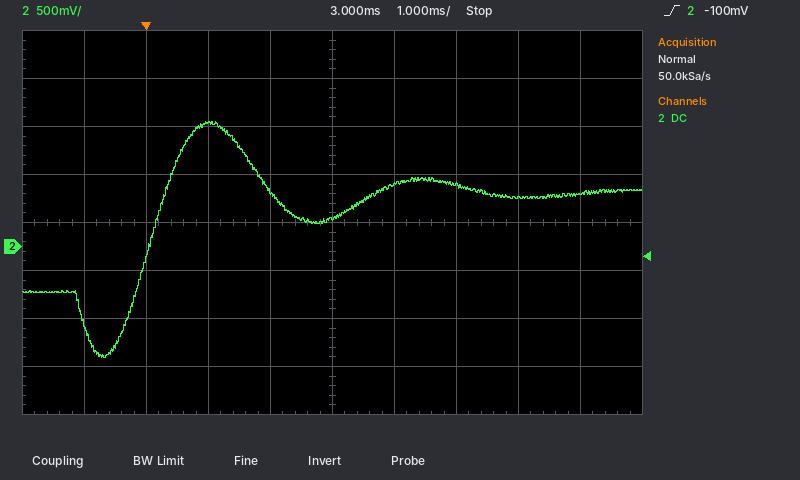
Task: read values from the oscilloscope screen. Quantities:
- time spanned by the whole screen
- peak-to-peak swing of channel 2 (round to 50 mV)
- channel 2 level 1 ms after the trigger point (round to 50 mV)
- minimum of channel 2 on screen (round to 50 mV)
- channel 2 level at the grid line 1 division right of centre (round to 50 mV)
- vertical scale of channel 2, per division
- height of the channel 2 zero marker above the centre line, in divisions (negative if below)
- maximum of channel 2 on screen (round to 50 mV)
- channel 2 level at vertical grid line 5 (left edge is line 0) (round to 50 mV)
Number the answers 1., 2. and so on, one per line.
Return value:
1. 10 ms
2. 2.45 V
3. 1.30 V
4. -1.15 V
5. 650 mV
6. 500 mV
7. -0.5 div
8. 1.30 V
9. 300 mV
